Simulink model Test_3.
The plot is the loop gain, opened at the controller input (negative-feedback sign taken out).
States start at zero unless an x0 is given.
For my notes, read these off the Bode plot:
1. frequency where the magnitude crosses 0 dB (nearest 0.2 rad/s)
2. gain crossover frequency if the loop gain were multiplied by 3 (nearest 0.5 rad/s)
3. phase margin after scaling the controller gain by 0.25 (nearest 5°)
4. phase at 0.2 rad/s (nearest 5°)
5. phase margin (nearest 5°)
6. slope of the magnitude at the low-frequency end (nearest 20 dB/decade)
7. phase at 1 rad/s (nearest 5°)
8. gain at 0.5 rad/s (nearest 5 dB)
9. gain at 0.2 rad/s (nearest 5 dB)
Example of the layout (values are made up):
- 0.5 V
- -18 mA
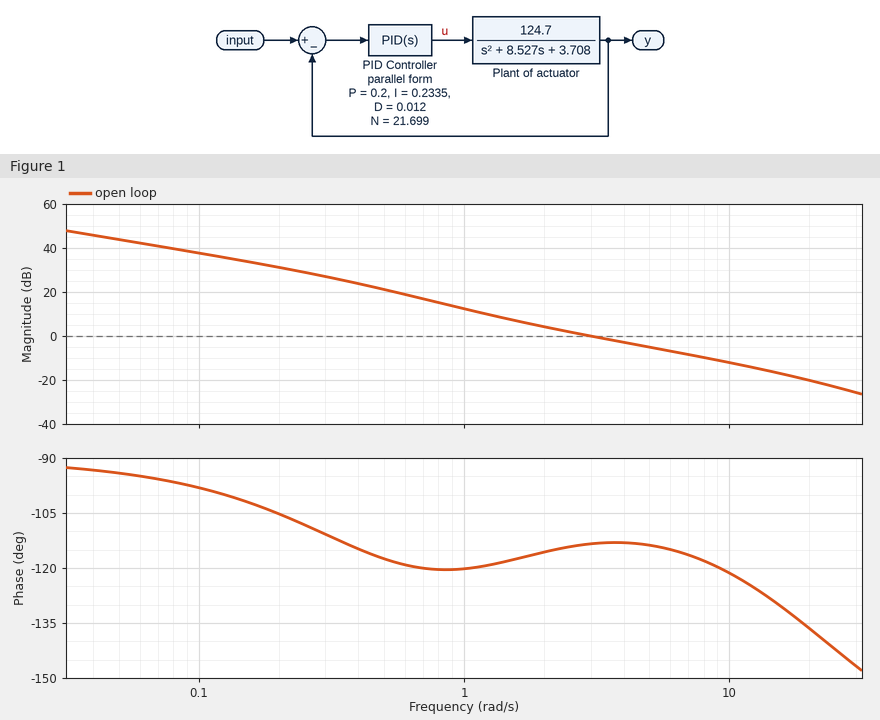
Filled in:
- 3.0 rad/s
- 8.0 rad/s
- 60°
- -105°
- 65°
- -20 dB/decade
- -120°
- 20 dB
- 30 dB
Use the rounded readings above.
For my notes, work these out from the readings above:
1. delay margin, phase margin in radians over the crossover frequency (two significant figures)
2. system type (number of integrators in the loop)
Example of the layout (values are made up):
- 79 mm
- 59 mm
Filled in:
- 0.38 s
- 1
